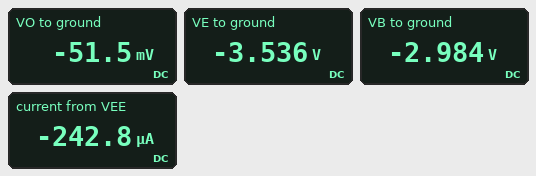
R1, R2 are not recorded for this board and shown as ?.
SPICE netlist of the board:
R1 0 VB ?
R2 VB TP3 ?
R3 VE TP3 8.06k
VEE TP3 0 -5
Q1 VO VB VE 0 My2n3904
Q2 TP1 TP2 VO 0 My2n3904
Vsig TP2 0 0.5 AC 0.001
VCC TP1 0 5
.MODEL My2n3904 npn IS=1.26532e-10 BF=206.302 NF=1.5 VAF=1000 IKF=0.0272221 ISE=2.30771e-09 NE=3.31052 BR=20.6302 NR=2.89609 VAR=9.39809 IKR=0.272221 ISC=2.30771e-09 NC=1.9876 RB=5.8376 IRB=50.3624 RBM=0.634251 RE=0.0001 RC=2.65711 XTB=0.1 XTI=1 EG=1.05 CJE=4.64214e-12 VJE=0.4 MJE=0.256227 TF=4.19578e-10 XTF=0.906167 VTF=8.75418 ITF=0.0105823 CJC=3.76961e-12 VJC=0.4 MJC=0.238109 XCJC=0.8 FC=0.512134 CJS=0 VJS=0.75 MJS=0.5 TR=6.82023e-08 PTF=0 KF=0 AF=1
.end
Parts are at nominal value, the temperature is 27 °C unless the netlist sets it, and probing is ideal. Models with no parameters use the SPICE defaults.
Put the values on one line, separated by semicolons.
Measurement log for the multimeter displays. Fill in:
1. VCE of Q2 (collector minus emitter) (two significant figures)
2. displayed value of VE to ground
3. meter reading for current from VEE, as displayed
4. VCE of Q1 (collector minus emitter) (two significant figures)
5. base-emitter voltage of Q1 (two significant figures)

5.1 V; -3.536 V; -242.8 µA; 3.5 V; 550 mV
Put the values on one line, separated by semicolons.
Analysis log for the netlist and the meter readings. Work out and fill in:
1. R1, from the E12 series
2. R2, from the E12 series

47 kΩ; 33 kΩ
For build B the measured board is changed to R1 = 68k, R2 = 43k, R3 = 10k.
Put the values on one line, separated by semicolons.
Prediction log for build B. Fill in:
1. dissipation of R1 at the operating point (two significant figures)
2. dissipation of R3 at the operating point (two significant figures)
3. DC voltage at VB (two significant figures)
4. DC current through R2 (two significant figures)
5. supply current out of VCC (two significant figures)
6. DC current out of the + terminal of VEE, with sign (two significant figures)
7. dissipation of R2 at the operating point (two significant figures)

140 µW; 180 µW; -3.1 V; 44 µA; 130 µA; -180 µA; 83 µW
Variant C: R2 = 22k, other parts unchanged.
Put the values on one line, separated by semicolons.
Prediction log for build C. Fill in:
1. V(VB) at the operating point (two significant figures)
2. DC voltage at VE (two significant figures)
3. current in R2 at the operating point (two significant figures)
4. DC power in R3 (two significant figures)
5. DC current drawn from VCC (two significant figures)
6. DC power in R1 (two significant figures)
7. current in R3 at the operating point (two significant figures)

-3.4 V; -4.0 V; 71 µA; 130 µW; 120 µA; 250 µW; 130 µA
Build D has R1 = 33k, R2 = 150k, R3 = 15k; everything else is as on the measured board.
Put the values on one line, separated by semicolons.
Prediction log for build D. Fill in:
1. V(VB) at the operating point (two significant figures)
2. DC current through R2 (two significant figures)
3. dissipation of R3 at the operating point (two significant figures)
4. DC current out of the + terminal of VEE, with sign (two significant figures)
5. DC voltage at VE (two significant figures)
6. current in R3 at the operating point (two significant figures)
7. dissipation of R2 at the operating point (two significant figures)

-980 mV; 27 µA; 800 µW; -260 µA; -1.5 V; 230 µA; 110 µW
